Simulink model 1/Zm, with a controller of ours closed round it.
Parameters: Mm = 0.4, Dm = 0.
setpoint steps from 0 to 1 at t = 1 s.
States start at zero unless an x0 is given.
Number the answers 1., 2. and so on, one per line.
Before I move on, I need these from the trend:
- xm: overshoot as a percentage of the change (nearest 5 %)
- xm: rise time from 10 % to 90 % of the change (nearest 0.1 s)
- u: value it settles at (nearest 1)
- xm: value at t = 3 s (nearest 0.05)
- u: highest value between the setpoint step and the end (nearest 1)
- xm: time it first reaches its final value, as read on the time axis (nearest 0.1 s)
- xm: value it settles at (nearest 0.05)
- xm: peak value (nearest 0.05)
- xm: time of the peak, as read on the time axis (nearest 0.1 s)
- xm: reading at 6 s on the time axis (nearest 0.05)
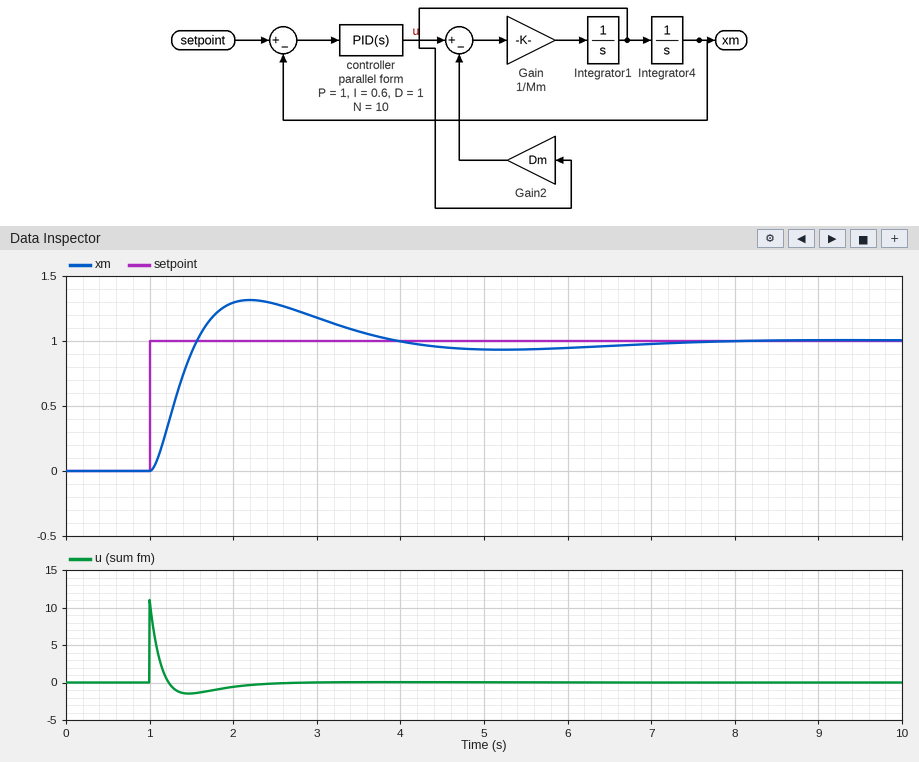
1. 30 %
2. 0.4 s
3. 0
4. 1.20
5. 11
6. 1.6 s
7. 1.00
8. 1.30
9. 2.2 s
10. 0.95
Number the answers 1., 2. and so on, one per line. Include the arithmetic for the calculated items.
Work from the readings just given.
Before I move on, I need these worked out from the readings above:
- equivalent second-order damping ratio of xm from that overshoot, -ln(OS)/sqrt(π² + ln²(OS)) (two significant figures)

1. ln(0.3) = -1.204; 1.204 / sqrt(9.870 + 1.450) = 0.36
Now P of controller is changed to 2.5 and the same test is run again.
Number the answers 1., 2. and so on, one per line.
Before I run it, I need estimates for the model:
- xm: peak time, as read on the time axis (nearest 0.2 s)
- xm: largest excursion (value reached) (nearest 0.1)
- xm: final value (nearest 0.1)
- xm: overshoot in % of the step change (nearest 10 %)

1. 1.8 s
2. 1.4
3. 1.0
4. 40 %
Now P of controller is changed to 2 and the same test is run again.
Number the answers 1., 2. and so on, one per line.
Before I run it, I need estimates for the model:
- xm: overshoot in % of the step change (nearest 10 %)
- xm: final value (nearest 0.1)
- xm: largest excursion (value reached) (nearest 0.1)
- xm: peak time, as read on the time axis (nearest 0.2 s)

1. 40 %
2. 1.0
3. 1.4
4. 2.0 s
